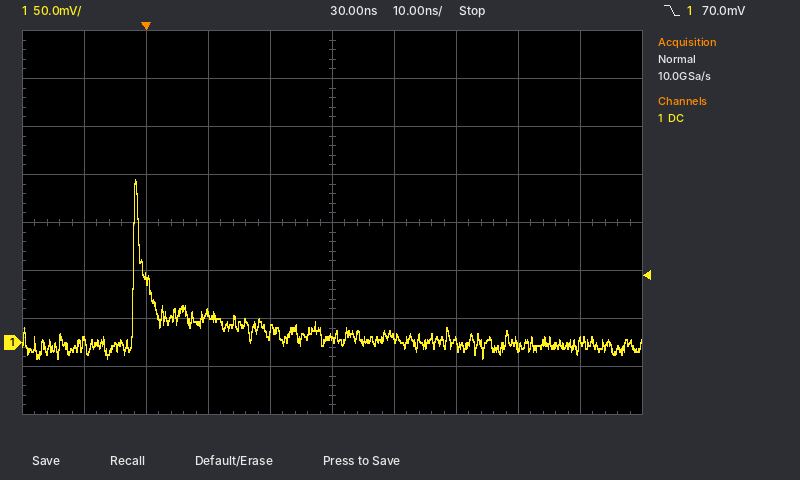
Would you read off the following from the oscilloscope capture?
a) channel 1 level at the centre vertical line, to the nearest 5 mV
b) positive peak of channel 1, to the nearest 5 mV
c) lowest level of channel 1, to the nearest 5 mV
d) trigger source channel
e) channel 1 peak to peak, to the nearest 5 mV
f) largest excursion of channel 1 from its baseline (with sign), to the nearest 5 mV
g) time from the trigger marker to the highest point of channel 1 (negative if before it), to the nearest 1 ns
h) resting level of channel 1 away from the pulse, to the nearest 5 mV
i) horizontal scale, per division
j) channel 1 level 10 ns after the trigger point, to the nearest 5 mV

5 mV
170 mV
-15 mV
channel 1
185 mV
+170 mV
-2 ns
0 mV
10 ns
30 mV
